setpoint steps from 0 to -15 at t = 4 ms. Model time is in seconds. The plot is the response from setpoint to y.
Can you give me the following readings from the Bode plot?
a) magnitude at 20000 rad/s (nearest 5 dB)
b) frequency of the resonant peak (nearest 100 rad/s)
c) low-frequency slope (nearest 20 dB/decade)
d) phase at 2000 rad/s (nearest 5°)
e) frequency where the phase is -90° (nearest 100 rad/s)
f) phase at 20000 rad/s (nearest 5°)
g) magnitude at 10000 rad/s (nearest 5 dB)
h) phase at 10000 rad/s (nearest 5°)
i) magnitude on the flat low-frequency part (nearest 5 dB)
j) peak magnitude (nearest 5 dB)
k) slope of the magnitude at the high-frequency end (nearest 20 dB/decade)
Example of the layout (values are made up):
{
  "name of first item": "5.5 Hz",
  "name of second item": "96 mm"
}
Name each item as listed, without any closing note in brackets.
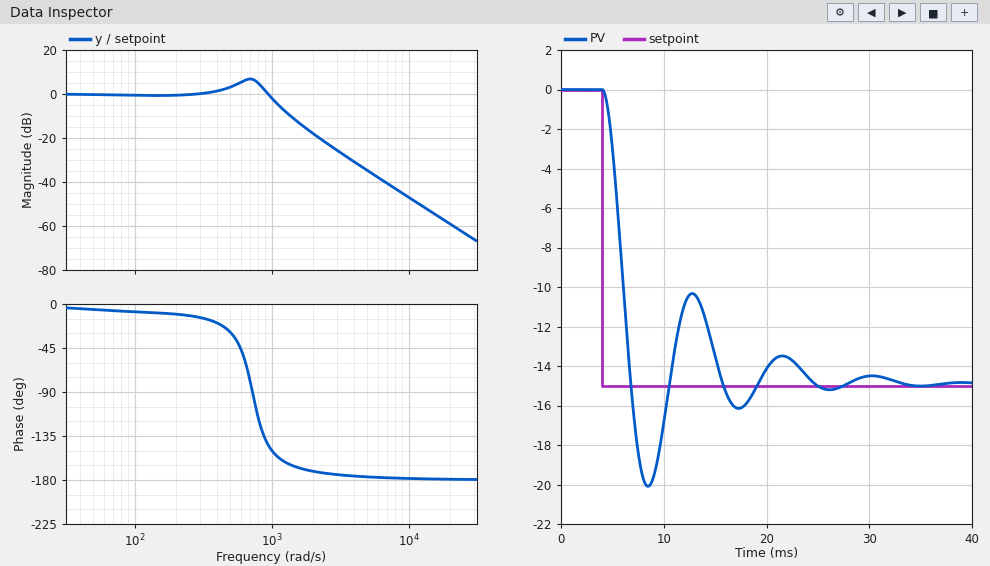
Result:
{
  "magnitude at 20000 rad/s": "-60 dB",
  "frequency of the resonant peak": "700 rad/s",
  "low-frequency slope": "0 dB/decade",
  "phase at 2000 rad/s": "-170°",
  "frequency where the phase is -90°": "700 rad/s",
  "phase at 20000 rad/s": "-180°",
  "magnitude at 10000 rad/s": "-45 dB",
  "phase at 10000 rad/s": "-180°",
  "magnitude on the flat low-frequency part": "0 dB",
  "peak magnitude": "5 dB",
  "slope of the magnitude at the high-frequency end": "-40 dB/decade"
}
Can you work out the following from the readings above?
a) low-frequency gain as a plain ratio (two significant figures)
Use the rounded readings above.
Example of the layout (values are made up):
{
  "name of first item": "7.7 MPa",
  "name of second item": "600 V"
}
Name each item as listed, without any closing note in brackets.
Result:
{
  "low-frequency gain as a plain ratio": "1.0"
}
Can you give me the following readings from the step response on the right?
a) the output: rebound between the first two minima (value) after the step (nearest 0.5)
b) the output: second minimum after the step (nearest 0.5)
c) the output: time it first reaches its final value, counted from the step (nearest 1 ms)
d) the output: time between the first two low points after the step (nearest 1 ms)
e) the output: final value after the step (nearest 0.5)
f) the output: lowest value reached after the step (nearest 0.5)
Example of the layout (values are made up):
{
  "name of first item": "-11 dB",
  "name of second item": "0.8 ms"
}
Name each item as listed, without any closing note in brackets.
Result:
{
  "the output: rebound between the first two minima (value) after the step": "-10.5",
  "the output: second minimum after the step": "-16.0",
  "the output: time it first reaches its final value, counted from the step": "3 ms",
  "the output: time between the first two low points after the step": "9 ms",
  "the output: final value after the step": "-15.0",
  "the output: lowest value reached after the step": "-20.0"
}
